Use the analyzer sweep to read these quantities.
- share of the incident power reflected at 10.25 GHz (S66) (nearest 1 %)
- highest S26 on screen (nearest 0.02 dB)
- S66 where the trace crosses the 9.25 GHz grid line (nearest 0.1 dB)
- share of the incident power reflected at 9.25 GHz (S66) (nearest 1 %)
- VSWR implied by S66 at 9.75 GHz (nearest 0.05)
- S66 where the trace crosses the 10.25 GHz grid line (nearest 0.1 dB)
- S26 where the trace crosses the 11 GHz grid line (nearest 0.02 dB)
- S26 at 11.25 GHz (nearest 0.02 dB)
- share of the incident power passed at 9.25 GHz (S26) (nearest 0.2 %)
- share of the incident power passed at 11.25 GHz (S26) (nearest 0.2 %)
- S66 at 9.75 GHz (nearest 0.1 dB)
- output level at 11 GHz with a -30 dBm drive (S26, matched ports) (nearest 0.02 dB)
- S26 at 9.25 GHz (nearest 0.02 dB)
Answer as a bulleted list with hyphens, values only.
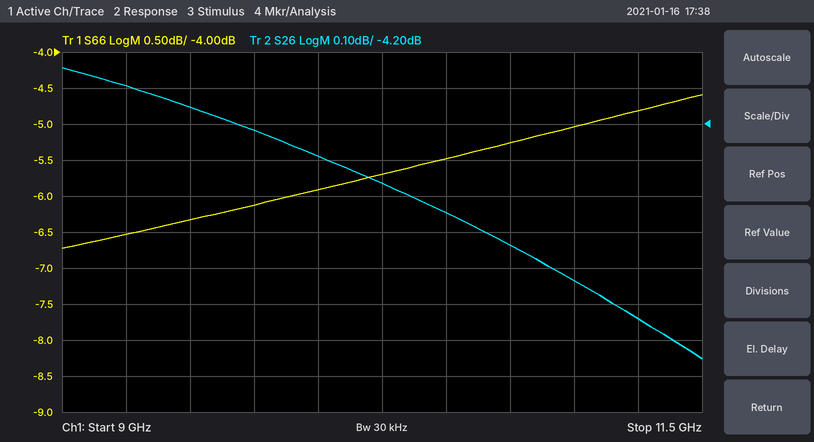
- 27 %
- -4.04 dB
- -6.5 dB
- 22 %
- 2.95
- -5.7 dB
- -4.64 dB
- -4.74 dB
- 39.0 %
- 33.6 %
- -6.1 dB
- -34.64 dBm
- -4.10 dB
